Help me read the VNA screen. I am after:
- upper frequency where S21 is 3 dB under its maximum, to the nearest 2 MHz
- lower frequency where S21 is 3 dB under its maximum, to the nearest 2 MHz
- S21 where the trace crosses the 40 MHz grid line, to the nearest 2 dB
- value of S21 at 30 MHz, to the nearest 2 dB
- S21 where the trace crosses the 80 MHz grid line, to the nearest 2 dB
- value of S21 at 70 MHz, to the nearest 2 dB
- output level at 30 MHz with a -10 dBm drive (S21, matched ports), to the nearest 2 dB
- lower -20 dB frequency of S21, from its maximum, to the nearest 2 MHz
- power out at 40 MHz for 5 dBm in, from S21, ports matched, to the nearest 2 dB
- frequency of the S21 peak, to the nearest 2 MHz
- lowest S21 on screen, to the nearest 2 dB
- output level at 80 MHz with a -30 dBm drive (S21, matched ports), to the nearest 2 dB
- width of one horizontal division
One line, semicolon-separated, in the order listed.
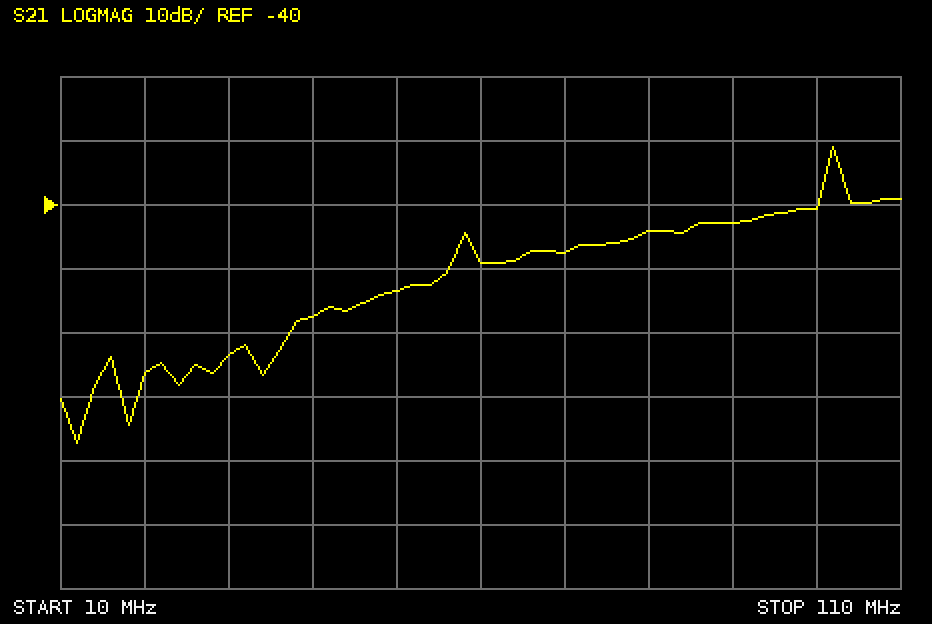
102 MHz; 102 MHz; -58 dB; -64 dB; -44 dB; -48 dB; -74 dBm; 56 MHz; -52 dBm; 102 MHz; -78 dB; -74 dBm; 10 MHz
